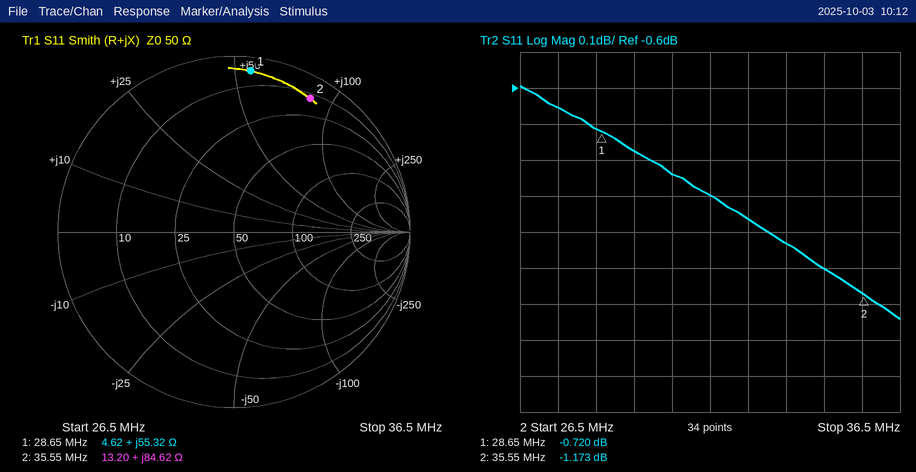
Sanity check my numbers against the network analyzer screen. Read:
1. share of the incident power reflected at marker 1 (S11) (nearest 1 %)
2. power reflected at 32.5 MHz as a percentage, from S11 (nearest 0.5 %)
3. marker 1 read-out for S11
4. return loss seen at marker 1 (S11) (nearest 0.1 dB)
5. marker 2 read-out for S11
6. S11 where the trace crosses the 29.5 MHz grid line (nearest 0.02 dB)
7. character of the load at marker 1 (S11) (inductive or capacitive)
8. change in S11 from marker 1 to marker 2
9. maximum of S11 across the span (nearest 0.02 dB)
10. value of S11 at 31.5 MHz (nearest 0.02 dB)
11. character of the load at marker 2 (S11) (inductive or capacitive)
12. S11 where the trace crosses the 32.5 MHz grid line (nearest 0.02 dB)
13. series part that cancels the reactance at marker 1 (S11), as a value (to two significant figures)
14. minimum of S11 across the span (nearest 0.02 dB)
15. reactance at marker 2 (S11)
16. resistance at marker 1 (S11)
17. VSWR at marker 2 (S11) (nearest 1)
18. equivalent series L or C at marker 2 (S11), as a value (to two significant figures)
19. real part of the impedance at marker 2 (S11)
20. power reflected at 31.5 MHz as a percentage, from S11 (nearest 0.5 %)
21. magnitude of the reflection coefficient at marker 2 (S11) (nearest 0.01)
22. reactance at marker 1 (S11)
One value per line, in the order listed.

85 %
80.0 %
-0.720 dB
0.7 dB
-1.173 dB
-0.78 dB
inductive
-0.453 dB
-0.60 dB
-0.90 dB
inductive
-0.96 dB
100 pF
-1.24 dB
+84.62 Ω
4.62 Ω
15
380 nH
13.20 Ω
81.5 %
0.87
+55.32 Ω
